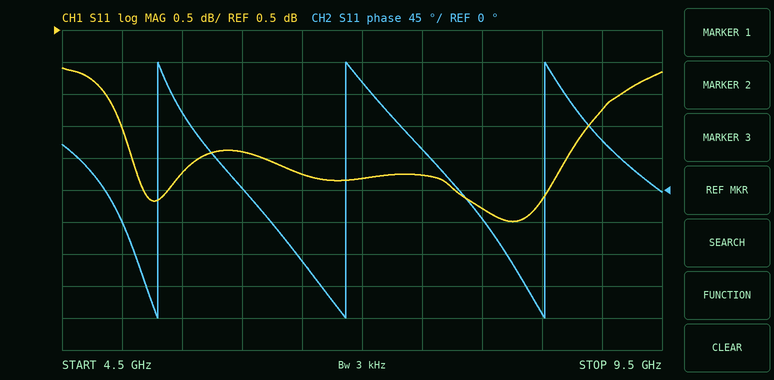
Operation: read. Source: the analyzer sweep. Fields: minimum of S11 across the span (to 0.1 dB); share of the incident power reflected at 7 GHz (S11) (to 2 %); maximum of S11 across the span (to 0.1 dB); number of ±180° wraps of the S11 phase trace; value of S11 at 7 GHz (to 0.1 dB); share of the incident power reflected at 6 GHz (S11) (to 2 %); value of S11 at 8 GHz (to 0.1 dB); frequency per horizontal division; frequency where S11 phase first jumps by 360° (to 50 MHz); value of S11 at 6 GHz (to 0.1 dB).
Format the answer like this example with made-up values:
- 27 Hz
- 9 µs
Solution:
- -2.5 dB
- 66 %
- -0.1 dB
- 3
- -1.8 dB
- 72 %
- -2.3 dB
- 500 MHz
- 5.30 GHz
- -1.4 dB
